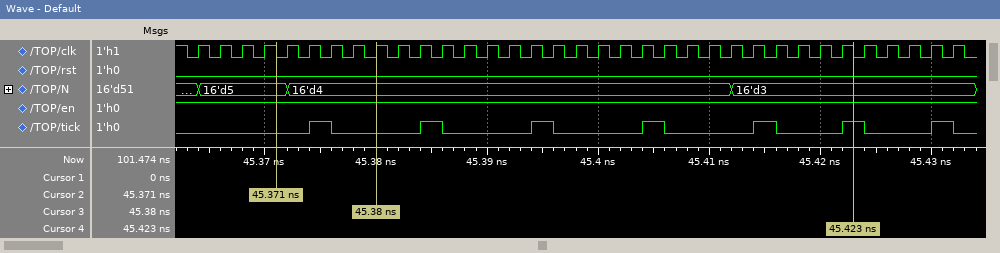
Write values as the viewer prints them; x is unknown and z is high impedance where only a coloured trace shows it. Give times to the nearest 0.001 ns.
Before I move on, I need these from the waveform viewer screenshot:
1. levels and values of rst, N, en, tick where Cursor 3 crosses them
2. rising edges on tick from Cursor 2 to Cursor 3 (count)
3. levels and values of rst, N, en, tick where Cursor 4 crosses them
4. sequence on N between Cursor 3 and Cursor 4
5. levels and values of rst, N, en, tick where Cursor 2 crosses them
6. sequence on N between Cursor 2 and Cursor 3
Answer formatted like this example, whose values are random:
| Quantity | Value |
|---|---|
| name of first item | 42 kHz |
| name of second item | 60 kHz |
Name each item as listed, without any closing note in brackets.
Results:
| Quantity | Value |
|---|---|
| levels and values of rst, N, en, tick where Cursor 3 crosses them | rst=0, N=16'd4, en=1, tick=0 |
| rising edges on tick from Cursor 2 to Cursor 3 | 1 |
| levels and values of rst, N, en, tick where Cursor 4 crosses them | rst=0, N=16'd3, en=1, tick=1 |
| sequence on N between Cursor 3 and Cursor 4 | 16'd4, 16'd3 |
| levels and values of rst, N, en, tick where Cursor 2 crosses them | rst=0, N=16'd5, en=1, tick=0 |
| sequence on N between Cursor 2 and Cursor 3 | 16'd5, 16'd4 |
